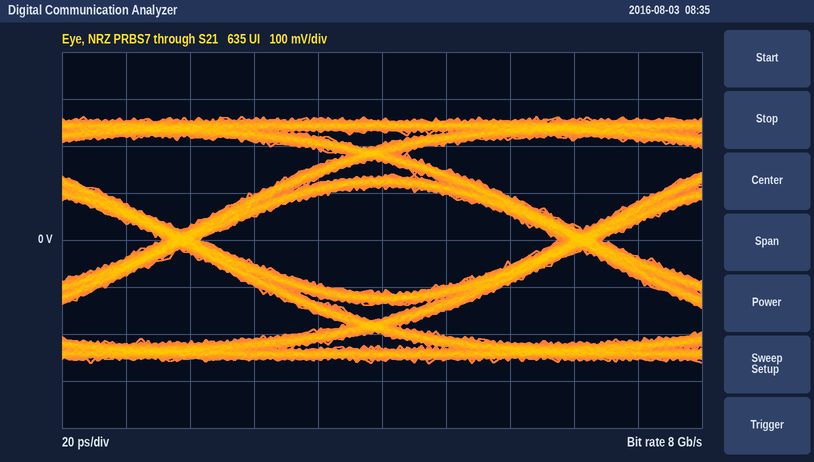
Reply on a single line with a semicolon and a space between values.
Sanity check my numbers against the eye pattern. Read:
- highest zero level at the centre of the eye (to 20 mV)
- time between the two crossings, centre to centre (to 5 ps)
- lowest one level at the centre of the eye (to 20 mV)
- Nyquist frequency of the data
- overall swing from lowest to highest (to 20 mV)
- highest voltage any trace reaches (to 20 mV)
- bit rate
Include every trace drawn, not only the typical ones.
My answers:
-120 mV; 125 ps; 120 mV; 4 GHz; 520 mV; 260 mV; 8 Gb/s
